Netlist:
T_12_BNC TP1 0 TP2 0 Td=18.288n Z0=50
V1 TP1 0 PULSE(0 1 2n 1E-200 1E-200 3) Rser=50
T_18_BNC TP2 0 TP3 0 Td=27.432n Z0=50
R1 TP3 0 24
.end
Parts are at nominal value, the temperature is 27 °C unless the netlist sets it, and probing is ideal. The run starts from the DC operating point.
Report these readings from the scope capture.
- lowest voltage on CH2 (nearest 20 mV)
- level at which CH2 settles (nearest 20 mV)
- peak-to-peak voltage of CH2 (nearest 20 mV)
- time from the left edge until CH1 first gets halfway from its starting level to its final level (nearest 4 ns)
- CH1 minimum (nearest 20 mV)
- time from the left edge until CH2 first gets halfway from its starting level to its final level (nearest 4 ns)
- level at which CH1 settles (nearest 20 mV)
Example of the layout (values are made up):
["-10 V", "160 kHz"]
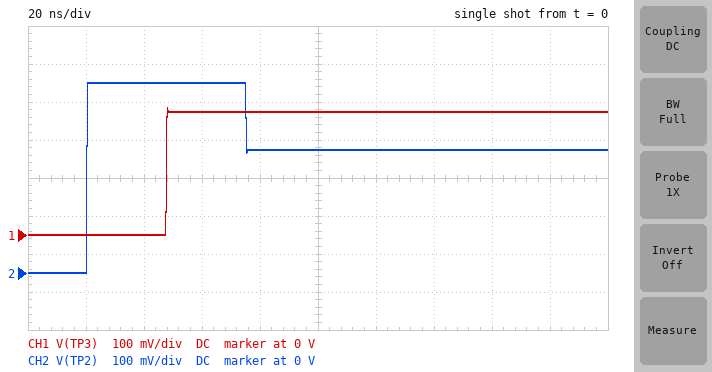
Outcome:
["0 V", "320 mV", "500 mV", "48 ns", "0 V", "20 ns", "320 mV"]
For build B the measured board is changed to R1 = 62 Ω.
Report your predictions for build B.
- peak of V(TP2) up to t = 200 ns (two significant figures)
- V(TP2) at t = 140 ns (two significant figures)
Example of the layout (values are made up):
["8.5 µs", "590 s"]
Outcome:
["560 mV", "550 mV"]
